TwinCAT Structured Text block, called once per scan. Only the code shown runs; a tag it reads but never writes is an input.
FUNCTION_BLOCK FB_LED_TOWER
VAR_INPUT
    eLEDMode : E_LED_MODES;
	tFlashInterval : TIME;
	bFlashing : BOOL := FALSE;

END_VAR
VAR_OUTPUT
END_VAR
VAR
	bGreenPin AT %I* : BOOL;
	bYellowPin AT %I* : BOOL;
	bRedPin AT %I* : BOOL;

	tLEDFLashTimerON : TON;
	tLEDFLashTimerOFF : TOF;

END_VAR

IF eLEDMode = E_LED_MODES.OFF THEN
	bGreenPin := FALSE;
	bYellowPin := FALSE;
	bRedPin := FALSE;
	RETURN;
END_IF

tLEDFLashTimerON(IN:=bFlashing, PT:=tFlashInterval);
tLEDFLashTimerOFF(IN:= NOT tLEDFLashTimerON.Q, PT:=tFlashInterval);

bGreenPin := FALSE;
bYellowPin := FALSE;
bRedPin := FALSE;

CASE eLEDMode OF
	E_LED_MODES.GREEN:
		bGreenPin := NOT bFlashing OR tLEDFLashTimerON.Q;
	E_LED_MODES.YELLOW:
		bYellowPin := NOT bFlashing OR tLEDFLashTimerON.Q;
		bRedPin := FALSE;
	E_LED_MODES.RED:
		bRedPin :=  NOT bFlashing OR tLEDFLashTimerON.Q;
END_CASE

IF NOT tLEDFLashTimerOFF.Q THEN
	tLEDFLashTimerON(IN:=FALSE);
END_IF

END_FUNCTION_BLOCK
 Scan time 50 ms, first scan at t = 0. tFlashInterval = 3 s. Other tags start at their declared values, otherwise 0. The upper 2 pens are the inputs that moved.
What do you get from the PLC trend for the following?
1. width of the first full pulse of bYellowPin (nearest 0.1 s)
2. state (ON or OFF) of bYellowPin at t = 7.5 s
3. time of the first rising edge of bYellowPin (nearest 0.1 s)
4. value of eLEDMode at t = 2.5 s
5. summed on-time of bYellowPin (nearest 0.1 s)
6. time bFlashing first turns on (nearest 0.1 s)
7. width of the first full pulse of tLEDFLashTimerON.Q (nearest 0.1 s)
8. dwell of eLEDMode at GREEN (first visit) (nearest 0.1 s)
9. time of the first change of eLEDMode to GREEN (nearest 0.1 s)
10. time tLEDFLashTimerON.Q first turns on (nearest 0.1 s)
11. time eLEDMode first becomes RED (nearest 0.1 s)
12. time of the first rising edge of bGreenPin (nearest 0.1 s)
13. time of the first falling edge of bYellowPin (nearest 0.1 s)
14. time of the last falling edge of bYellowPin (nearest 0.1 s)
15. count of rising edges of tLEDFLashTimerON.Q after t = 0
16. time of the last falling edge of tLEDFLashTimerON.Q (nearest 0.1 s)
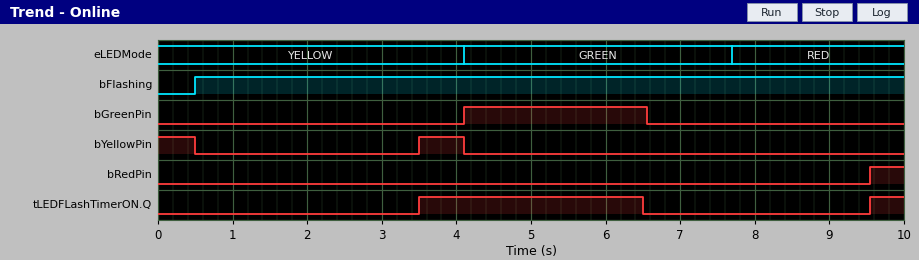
0.6 s
OFF
3.5 s
YELLOW
1.1 s
0.5 s
3.0 s
3.6 s
4.1 s
3.5 s
7.7 s
4.1 s
0.5 s
4.1 s
2
6.5 s
